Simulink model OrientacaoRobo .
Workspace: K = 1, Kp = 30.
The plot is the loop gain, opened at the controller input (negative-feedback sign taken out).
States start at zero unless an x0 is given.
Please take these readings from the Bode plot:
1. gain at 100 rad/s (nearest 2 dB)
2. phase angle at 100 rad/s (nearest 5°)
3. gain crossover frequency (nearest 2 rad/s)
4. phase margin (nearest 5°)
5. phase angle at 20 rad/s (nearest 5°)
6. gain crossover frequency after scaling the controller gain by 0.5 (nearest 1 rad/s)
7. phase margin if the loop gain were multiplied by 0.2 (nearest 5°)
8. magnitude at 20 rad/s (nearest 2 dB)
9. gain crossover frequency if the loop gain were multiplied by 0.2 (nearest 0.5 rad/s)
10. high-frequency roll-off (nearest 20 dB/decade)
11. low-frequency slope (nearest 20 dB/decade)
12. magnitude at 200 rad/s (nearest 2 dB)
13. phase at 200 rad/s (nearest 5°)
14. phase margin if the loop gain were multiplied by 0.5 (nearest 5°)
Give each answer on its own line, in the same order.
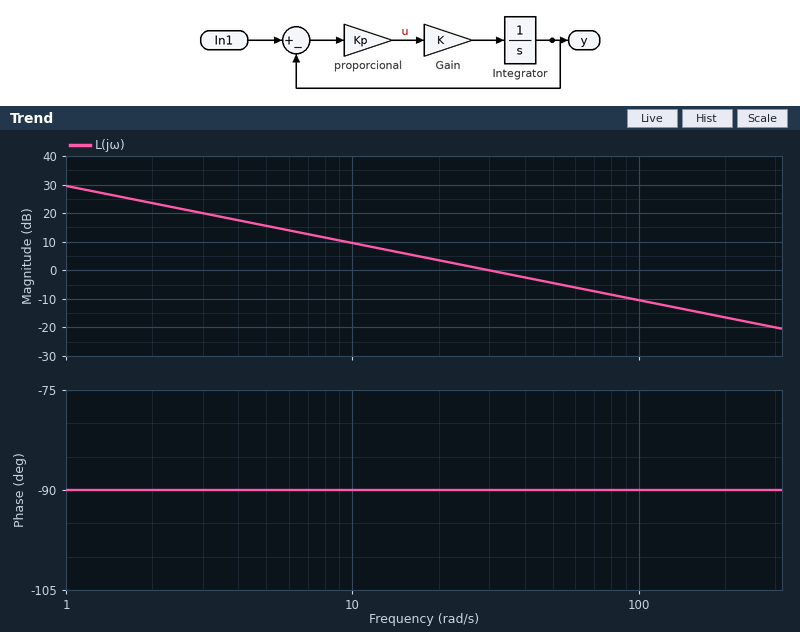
-10 dB
-90°
30 rad/s
90°
-90°
15 rad/s
90°
4 dB
6.0 rad/s
-20 dB/decade
-20 dB/decade
-16 dB
-90°
90°
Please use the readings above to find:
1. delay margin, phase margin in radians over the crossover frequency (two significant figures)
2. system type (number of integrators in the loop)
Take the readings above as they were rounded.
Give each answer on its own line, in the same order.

0.052 s
1
